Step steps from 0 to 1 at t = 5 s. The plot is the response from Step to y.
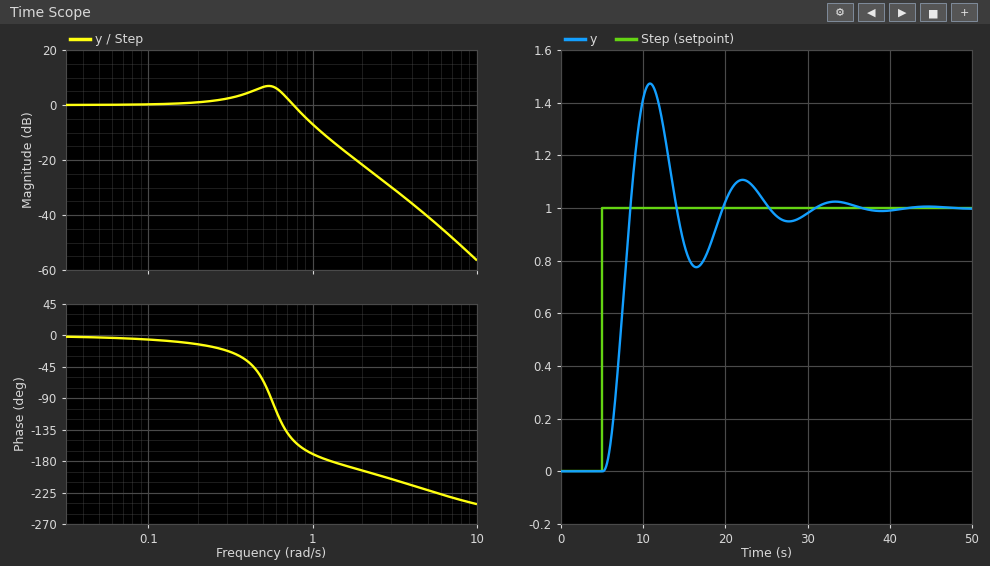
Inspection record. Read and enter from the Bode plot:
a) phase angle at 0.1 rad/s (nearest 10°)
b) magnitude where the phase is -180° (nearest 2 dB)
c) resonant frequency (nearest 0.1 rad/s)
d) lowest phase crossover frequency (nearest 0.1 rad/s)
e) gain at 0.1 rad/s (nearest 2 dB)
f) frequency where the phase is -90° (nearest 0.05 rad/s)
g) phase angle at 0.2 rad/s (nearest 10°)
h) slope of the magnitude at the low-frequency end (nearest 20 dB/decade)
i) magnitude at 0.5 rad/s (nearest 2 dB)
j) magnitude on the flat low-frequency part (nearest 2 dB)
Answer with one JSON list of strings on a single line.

["-10°", "-12 dB", "0.5 rad/s", "1.3 rad/s", "0 dB", "0.55 rad/s", "-10°", "0 dB/decade", "6 dB", "0 dB"]
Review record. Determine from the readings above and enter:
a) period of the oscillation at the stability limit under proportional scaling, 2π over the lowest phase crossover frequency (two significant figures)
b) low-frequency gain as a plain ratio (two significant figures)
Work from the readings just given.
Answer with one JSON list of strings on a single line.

["4.8 s", "1.0"]
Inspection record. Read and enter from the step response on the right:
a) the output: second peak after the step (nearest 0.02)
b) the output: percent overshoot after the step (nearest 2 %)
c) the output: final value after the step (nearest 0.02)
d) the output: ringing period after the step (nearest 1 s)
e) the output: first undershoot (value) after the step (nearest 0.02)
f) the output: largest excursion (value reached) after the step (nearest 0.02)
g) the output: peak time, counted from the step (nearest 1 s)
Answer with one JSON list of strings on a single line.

["1.10", "48 %", "1.00", "11 s", "0.78", "1.48", "6 s"]
